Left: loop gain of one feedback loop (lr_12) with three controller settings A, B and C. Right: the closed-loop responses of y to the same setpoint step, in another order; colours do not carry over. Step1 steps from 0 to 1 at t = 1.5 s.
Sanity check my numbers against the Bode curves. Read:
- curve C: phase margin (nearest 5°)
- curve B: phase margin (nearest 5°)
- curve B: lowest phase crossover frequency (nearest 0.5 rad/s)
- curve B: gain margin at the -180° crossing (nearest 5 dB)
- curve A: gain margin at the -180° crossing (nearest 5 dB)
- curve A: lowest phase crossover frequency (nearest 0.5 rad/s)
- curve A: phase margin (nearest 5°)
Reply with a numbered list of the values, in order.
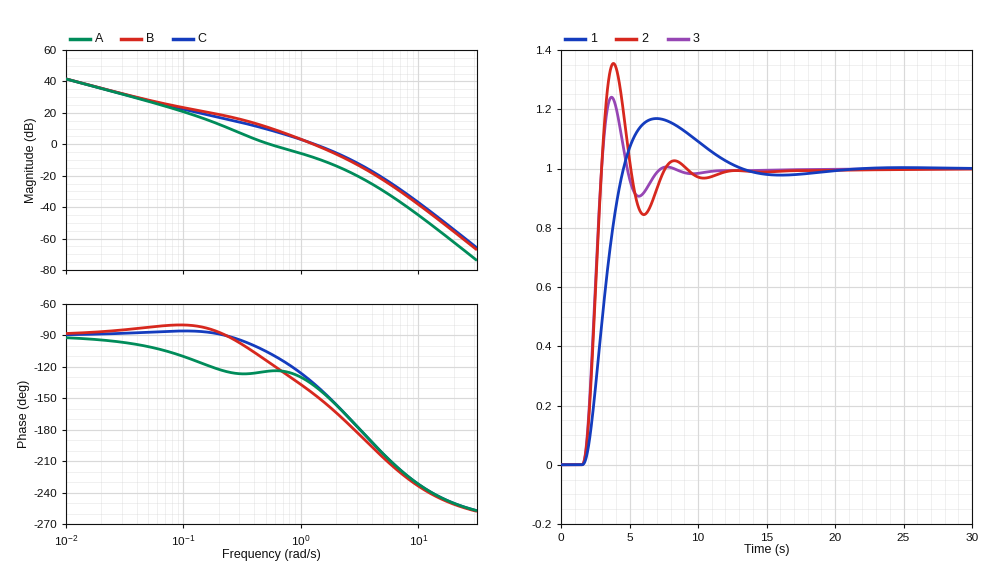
1. 45°
2. 35°
3. 3.0 rad/s
4. 10 dB
5. 20 dB
6. 3.0 rad/s
7. 55°
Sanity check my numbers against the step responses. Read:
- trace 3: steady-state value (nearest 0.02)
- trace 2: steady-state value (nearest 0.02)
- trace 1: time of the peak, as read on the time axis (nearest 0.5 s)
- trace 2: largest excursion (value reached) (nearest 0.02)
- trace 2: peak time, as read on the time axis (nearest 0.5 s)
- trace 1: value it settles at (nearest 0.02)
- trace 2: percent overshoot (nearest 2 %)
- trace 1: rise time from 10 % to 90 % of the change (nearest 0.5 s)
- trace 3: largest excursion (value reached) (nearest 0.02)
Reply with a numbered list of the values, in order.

1. 1.00
2. 1.00
3. 7.0 s
4. 1.36
5. 4.0 s
6. 1.00
7. 36 %
8. 2.0 s
9. 1.24
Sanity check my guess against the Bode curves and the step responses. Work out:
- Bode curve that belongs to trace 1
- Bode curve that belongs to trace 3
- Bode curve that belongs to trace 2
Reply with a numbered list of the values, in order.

1. A
2. C
3. B
